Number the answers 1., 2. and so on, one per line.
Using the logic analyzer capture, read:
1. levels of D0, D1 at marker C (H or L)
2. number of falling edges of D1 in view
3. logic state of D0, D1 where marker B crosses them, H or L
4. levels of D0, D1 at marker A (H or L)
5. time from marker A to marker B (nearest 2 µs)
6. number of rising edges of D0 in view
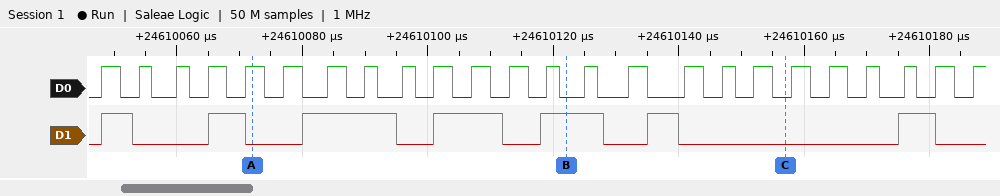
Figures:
1. D0=L, D1=L
2. 7
3. D0=L, D1=H
4. D0=H, D1=L
5. 50 µs
6. 24
